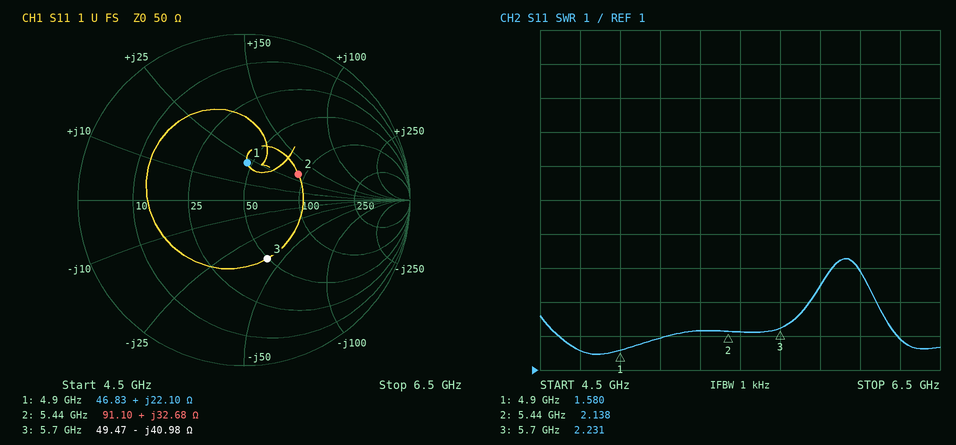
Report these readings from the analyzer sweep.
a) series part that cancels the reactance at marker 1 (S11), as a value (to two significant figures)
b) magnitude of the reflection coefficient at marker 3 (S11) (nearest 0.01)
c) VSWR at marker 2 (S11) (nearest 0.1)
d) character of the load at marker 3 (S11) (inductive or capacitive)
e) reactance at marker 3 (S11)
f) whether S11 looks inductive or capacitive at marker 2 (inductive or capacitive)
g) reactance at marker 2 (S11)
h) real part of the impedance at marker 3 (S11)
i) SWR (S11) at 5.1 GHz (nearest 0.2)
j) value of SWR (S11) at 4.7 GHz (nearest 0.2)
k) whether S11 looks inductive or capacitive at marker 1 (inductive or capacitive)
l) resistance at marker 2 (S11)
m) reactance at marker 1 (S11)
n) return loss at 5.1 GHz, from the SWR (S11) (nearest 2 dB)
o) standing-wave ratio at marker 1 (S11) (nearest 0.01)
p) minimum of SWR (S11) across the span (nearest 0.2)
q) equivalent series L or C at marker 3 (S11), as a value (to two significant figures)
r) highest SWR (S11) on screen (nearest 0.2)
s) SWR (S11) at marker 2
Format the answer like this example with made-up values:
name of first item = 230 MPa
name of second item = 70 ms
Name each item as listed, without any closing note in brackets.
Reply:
series part that cancels the reactance at marker 1 (S11), as a value = 1.5 pF
magnitude of the reflection coefficient at marker 3 (S11) = 0.38
VSWR at marker 2 (S11) = 2.1
character of the load at marker 3 (S11) = capacitive
reactance at marker 3 = -40.98 Ω
whether S11 looks inductive or capacitive at marker 2 = inductive
reactance at marker 2 = +32.68 Ω
real part of the impedance at marker 3 = 49.47 Ω
SWR (S11) at 5.1 GHz = 2.0
value of SWR (S11) at 4.7 GHz = 1.6
whether S11 looks inductive or capacitive at marker 1 = inductive
resistance at marker 2 = 91.10 Ω
reactance at marker 1 = +22.10 Ω
return loss at 5.1 GHz, from the SWR (S11) = 10 dB
standing-wave ratio at marker 1 (S11) = 1.58
minimum of SWR (S11) across the span = 1.4
equivalent series L or C at marker 3 (S11), as a value = 680 fF
highest SWR (S11) on screen = 4.2
SWR (S11) at marker 2 = 2.138
